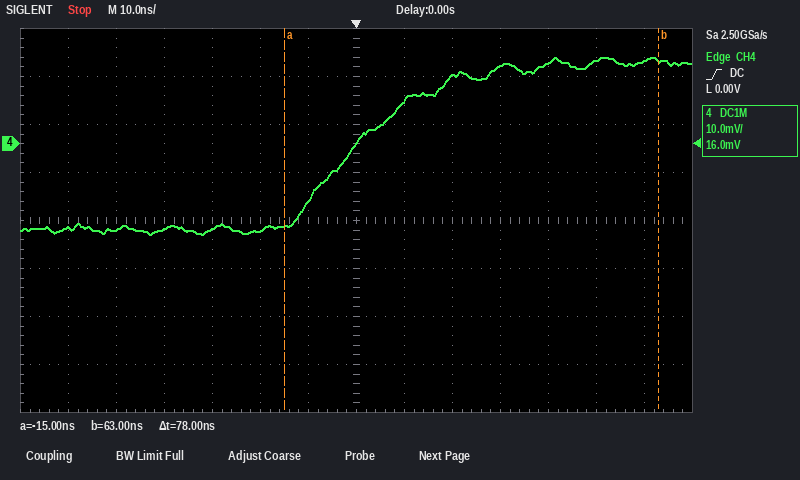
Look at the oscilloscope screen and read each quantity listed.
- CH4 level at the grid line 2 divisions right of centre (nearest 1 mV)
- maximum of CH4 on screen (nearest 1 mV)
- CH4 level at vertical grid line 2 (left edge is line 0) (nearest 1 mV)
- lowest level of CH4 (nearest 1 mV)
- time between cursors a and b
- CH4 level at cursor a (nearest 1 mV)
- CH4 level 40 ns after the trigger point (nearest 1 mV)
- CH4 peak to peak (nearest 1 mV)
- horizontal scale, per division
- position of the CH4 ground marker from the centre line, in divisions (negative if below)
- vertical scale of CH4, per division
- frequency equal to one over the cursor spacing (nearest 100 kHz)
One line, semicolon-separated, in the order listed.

14 mV; 18 mV; -18 mV; -19 mV; 78 ns; -17 mV; 17 mV; 37 mV; 10 ns; +1.6 div; 10 mV; 12.8 MHz
